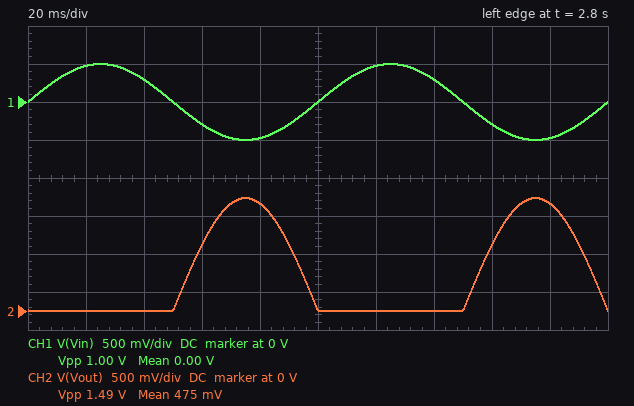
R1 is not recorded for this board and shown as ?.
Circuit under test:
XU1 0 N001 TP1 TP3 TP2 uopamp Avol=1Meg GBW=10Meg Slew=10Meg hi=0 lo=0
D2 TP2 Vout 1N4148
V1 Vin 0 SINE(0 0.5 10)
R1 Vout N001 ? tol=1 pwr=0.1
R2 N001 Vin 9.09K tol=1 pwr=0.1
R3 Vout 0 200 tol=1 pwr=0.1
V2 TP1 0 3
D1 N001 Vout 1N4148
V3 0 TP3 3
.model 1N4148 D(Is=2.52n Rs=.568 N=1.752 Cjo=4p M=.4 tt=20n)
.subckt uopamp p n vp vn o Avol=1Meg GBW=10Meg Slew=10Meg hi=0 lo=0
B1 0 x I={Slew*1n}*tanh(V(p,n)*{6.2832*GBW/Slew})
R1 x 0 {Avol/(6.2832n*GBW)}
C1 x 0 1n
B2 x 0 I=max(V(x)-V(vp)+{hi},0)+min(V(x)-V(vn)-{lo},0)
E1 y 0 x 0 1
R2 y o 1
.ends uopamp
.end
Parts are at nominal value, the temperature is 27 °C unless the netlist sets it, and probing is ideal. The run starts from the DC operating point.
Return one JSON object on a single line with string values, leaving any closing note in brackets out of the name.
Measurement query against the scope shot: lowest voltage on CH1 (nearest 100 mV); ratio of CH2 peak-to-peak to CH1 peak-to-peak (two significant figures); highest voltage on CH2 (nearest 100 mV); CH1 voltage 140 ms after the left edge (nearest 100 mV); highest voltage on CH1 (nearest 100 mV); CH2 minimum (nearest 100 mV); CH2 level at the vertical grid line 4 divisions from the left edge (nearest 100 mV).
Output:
{"lowest voltage on CH1": "-500 mV", "ratio of CH2 peak-to-peak to CH1 peak-to-peak": "1.5", "highest voltage on CH2": "1.5 V", "CH1 voltage 140 ms after the left edge": "300 mV", "highest voltage on CH1": "500 mV", "CH2 minimum": "0 V", "CH2 level at the vertical grid line 4 divisions from the left edge": "1.4 V"}
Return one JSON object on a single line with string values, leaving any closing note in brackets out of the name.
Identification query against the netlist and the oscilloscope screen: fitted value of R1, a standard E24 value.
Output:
{"fitted value of R1, a standard E24 value": "27 kΩ"}
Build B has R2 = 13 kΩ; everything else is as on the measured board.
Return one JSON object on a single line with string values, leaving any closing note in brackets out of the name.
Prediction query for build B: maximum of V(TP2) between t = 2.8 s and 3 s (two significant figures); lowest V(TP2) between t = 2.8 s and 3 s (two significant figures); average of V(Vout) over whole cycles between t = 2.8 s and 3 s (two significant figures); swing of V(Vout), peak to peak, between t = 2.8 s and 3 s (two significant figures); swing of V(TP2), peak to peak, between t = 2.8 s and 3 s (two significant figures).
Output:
{"maximum of V(TP2) between t = 2.8 s and 3 s": "1.7 V", "lowest V(TP2) between t = 2.8 s and 3 s": "-3.0 V", "average of V(Vout) over whole cycles between t = 2.8 s and 3 s": "330 mV", "swing of V(Vout), peak to peak, between t = 2.8 s and 3 s": "1.0 V", "swing of V(TP2), peak to peak, between t = 2.8 s and 3 s": "4.7 V"}
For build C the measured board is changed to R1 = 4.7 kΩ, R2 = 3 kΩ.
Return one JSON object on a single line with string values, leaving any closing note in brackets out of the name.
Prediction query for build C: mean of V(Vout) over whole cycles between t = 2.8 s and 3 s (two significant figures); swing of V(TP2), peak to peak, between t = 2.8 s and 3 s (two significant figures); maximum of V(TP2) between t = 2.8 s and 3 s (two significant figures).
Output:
{"mean of V(Vout) over whole cycles between t = 2.8 s and 3 s": "250 mV", "swing of V(TP2), peak to peak, between t = 2.8 s and 3 s": "4.4 V", "maximum of V(TP2) between t = 2.8 s and 3 s": "1.4 V"}
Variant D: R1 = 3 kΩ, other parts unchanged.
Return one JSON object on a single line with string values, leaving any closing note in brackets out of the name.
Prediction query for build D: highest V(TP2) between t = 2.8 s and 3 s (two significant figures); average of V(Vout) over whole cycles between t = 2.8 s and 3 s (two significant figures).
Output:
{"highest V(TP2) between t = 2.8 s and 3 s": "740 mV", "average of V(Vout) over whole cycles between t = 2.8 s and 3 s": "55 mV"}
